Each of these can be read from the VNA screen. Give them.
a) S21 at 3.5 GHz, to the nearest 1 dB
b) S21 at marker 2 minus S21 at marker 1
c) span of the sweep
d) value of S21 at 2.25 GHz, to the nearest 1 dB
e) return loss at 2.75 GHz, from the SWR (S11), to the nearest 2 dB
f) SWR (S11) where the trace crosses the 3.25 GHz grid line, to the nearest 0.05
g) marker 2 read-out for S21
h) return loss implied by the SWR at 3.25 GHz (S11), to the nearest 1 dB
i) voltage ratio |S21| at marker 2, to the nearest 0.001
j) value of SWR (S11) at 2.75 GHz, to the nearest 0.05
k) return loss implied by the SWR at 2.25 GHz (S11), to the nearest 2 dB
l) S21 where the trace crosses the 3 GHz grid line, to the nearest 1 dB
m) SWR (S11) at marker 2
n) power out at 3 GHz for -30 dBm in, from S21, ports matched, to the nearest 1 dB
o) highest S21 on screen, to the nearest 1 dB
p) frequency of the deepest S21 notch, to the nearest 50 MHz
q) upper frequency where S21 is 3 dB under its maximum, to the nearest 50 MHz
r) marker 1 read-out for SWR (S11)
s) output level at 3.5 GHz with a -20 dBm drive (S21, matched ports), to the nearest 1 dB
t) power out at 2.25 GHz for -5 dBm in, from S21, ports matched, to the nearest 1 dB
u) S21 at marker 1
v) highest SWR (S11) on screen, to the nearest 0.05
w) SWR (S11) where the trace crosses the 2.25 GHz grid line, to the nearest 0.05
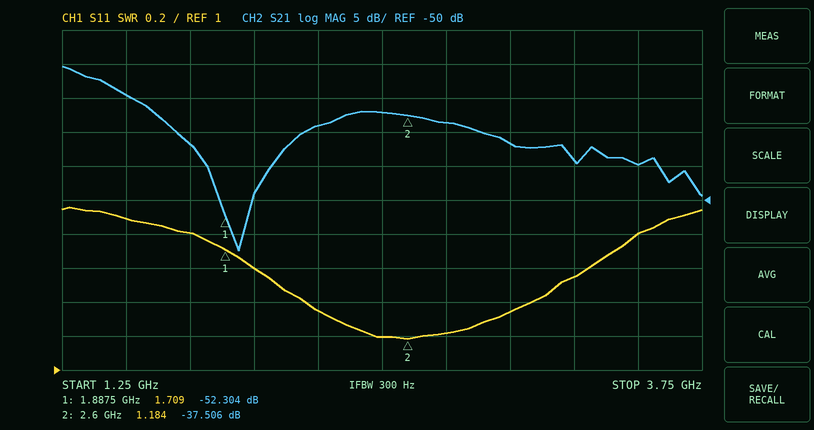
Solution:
-45 dB
14.798 dB
2.5 GHz
-39 dB
20 dB
1.55
-37.506 dB
13 dB
0.013
1.20
16 dB
-42 dB
1.184
-72 dBm
-30 dB
1.95 GHz
1.45 GHz
1.709
-65 dBm
-44 dBm
-52.304 dB
1.95
1.35
